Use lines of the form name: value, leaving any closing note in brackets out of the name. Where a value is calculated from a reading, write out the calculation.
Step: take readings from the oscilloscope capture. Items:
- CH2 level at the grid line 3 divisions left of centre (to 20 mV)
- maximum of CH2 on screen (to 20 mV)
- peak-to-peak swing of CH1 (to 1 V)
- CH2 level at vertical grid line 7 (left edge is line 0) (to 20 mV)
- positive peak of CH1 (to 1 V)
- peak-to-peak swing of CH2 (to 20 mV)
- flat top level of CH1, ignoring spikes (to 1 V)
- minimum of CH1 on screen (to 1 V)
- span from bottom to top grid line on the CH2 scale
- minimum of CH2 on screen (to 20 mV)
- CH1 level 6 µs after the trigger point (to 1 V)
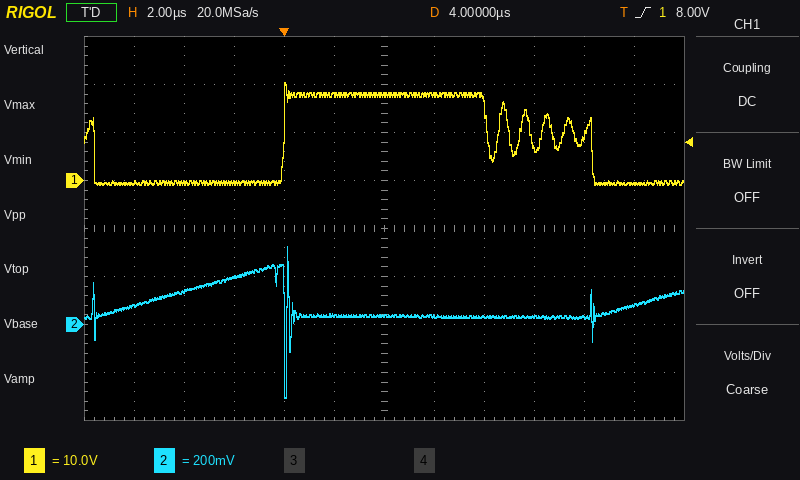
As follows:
CH2 level at the grid line 3 divisions left of centre: 200 mV
maximum of CH2 on screen: 320 mV
peak-to-peak swing of CH1: 20 V − (-1 V) = 21 V
CH2 level at vertical grid line 7 (left edge is line 0): 40 mV
positive peak of CH1: 20 V
peak-to-peak swing of CH2: 320 mV − (-300 mV) = 620 mV
flat top level of CH1, ignoring spikes: 18 V
minimum of CH1 on screen: -1 V
span from bottom to top grid line on the CH2 scale: 1.6 V
minimum of CH2 on screen: -300 mV
CH1 level 6 µs after the trigger point: 18 V
